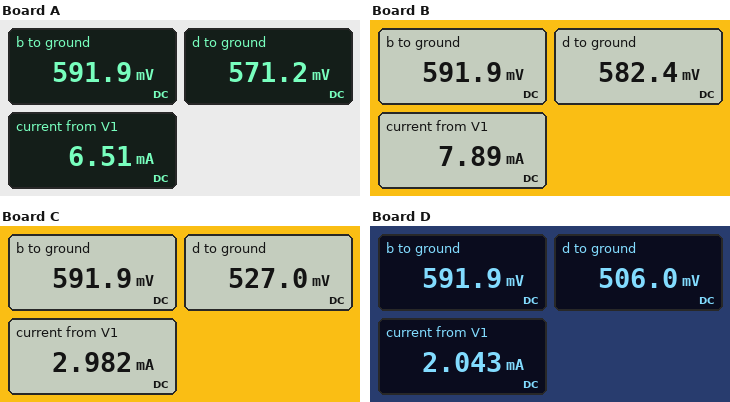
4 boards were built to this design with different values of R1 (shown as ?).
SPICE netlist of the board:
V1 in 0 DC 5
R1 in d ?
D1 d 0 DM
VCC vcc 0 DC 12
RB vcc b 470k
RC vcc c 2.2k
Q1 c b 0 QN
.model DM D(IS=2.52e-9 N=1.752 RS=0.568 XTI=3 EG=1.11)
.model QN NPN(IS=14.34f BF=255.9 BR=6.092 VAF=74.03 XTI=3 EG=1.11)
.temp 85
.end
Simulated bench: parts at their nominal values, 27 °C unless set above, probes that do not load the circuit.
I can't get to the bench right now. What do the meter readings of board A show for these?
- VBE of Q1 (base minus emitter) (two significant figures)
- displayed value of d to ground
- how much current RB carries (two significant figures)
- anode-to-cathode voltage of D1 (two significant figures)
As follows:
590 mV
571.2 mV
24 µA
570 mV
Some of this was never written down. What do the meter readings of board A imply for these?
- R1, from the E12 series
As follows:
680 Ω
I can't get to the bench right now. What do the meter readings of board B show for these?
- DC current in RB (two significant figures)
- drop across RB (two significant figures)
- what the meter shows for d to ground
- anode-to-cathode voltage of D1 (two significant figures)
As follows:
24 µA
11 V
582.4 mV
580 mV
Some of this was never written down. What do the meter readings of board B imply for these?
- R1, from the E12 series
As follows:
560 Ω
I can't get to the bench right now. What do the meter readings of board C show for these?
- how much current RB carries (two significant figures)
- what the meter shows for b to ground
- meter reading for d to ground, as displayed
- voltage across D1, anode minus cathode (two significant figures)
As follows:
24 µA
591.9 mV
527.0 mV
530 mV
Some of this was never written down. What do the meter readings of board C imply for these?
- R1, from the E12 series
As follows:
1.5 kΩ
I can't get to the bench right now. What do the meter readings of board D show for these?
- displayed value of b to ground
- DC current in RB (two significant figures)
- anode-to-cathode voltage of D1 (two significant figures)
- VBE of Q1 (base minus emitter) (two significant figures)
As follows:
591.9 mV
24 µA
510 mV
590 mV
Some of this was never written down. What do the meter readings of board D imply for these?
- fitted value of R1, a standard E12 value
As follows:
2.2 kΩ
